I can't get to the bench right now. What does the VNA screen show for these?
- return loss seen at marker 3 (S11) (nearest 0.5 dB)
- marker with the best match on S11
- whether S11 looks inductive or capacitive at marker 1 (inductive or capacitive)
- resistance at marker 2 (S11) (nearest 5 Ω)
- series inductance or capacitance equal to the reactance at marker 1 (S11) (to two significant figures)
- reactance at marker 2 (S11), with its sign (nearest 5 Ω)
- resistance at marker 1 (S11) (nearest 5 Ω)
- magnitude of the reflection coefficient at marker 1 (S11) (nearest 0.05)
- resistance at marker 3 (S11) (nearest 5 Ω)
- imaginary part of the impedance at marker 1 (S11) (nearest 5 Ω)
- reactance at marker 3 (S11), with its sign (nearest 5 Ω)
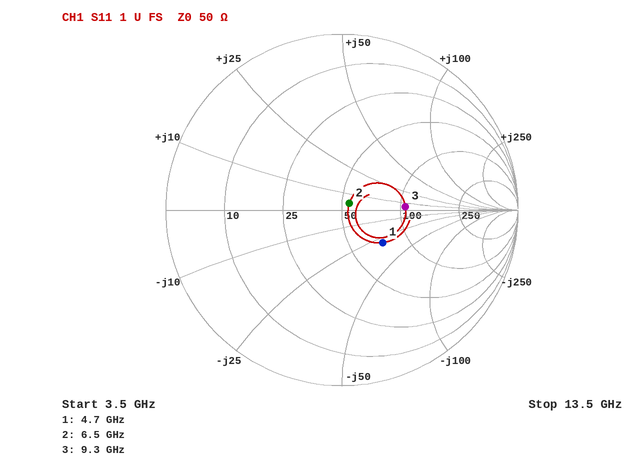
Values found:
9.0 dB
marker 2
capacitive
55 Ω
1.1 pF
+5 Ω
75 Ω
0.30
105 Ω
-30 Ω
+5 Ω
